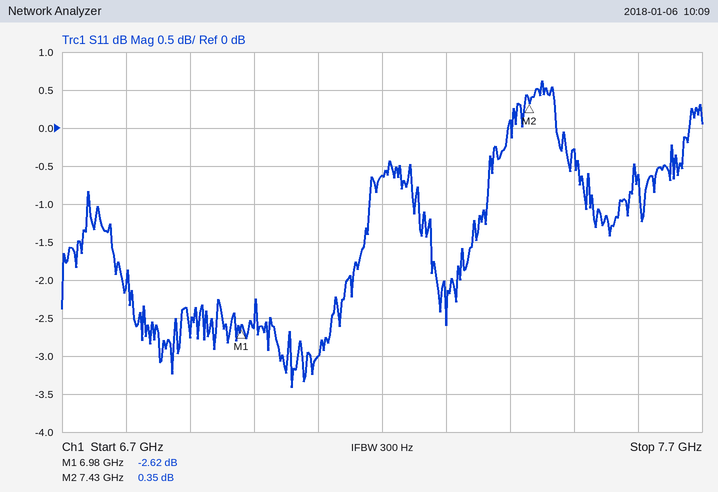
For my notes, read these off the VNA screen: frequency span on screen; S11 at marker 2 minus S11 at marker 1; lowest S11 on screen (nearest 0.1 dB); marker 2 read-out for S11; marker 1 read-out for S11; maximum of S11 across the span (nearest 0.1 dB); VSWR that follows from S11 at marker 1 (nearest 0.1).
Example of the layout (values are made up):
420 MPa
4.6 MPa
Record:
1 GHz
2.97 dB
-3.4 dB
0.35 dB
-2.62 dB
0.6 dB
6.7
